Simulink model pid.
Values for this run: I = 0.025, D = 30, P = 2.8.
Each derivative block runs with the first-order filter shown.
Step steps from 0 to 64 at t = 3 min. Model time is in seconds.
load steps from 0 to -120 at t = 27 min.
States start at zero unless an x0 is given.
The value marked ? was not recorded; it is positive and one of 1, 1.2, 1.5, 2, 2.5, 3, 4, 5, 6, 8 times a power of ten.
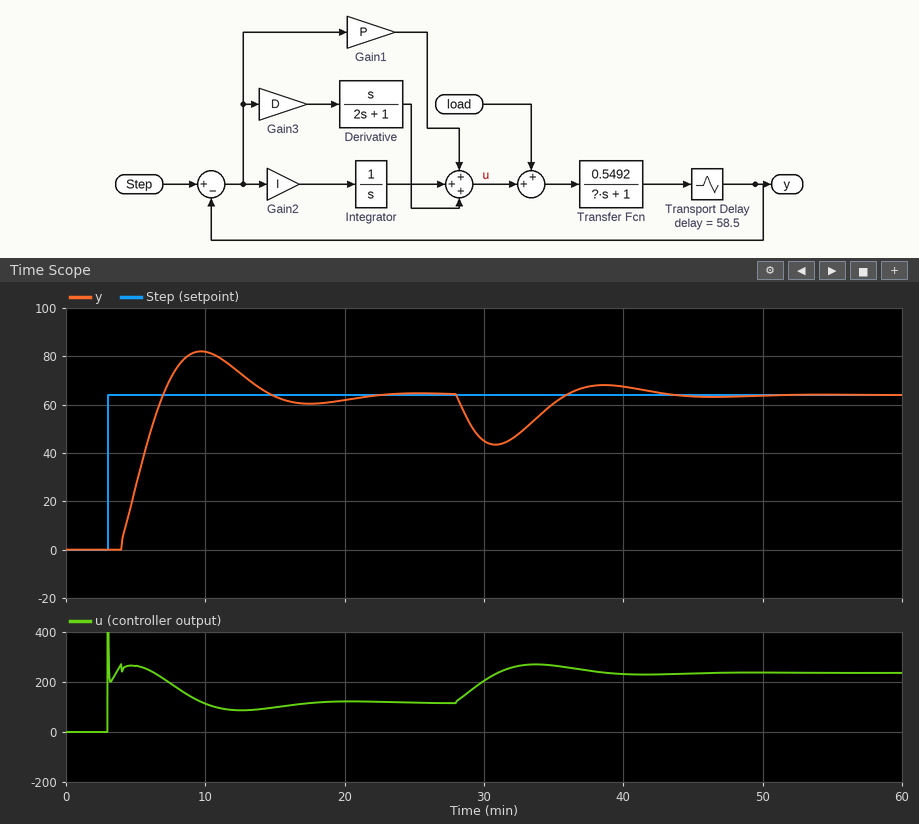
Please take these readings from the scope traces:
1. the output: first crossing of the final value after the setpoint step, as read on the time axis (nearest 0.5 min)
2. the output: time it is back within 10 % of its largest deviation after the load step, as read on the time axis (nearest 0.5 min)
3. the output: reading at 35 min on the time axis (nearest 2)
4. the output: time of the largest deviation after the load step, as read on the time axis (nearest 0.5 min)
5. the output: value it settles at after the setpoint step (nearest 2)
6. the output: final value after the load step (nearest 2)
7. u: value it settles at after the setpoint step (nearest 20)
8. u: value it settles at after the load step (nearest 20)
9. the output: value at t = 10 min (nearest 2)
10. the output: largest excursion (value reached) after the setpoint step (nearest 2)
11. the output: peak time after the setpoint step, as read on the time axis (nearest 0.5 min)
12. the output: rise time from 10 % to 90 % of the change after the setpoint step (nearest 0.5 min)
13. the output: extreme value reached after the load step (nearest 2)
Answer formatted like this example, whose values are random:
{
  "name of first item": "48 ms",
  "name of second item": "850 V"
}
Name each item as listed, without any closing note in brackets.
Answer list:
{
  "the output: first crossing of the final value after the setpoint step, as read on the time axis": "7.0 min",
  "the output: time it is back within 10 % of its largest deviation after the load step, as read on the time axis": "41.5 min",
  "the output: reading at 35 min on the time axis": "60",
  "the output: time of the largest deviation after the load step, as read on the time axis": "31.0 min",
  "the output: value it settles at after the setpoint step": "64",
  "the output: final value after the load step": "64",
  "u: value it settles at after the setpoint step": "120",
  "u: value it settles at after the load step": "240",
  "the output: value at t = 10 min": "82",
  "the output: largest excursion (value reached) after the setpoint step": "82",
  "the output: peak time after the setpoint step, as read on the time axis": "9.5 min",
  "the output: rise time from 10 % to 90 % of the change after the setpoint step": "2.5 min",
  "the output: extreme value reached after the load step": "44"
}
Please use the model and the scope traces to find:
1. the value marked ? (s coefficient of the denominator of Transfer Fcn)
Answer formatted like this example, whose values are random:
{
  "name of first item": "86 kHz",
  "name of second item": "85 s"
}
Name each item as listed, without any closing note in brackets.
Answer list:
{
  "the value marked ?": "300"
}
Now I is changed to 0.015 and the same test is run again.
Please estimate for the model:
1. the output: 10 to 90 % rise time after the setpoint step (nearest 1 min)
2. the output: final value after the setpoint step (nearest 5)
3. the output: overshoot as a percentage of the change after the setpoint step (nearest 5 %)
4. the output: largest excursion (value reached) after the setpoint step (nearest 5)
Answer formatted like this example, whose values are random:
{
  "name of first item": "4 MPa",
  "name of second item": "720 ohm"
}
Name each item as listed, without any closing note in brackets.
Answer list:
{
  "the output: 10 to 90 % rise time after the setpoint step": "3 min",
  "the output: final value after the setpoint step": "65",
  "the output: overshoot as a percentage of the change after the setpoint step": "10 %",
  "the output: largest excursion (value reached) after the setpoint step": "70"
}
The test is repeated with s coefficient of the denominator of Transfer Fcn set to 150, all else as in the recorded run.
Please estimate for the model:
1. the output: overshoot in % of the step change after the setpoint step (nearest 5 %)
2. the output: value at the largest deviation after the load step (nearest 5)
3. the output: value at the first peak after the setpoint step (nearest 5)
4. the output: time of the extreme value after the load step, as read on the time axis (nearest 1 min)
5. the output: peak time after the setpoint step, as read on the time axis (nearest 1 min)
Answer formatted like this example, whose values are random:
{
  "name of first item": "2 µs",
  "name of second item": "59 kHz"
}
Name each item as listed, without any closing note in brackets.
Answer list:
{
  "the output: overshoot in % of the step change after the setpoint step": "15 %",
  "the output: value at the largest deviation after the load step": "35",
  "the output: value at the first peak after the setpoint step": "75",
  "the output: time of the extreme value after the load step, as read on the time axis": "30 min",
  "the output: peak time after the setpoint step, as read on the time axis": "7 min"
}
